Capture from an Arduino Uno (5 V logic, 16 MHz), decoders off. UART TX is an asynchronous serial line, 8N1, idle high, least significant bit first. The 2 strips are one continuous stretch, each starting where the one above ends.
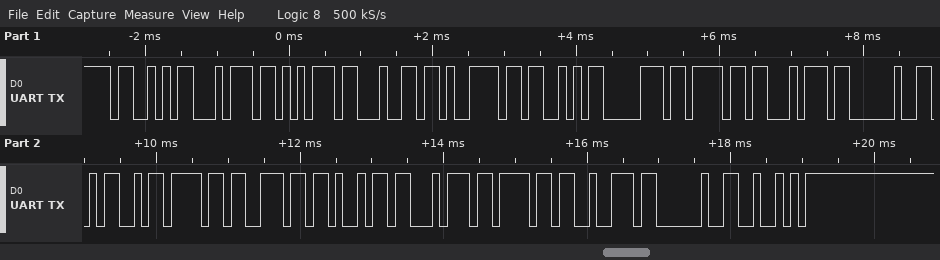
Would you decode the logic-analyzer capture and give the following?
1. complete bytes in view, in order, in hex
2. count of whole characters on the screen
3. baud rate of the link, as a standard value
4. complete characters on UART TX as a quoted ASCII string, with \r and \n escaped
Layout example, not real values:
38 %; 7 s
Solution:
53 74 75 64 79 53 70 6F 74 20 4D 6F 6E 69 74 6F 72 20 52; 19; 9600 baud; "StudySpot Monitor R"
